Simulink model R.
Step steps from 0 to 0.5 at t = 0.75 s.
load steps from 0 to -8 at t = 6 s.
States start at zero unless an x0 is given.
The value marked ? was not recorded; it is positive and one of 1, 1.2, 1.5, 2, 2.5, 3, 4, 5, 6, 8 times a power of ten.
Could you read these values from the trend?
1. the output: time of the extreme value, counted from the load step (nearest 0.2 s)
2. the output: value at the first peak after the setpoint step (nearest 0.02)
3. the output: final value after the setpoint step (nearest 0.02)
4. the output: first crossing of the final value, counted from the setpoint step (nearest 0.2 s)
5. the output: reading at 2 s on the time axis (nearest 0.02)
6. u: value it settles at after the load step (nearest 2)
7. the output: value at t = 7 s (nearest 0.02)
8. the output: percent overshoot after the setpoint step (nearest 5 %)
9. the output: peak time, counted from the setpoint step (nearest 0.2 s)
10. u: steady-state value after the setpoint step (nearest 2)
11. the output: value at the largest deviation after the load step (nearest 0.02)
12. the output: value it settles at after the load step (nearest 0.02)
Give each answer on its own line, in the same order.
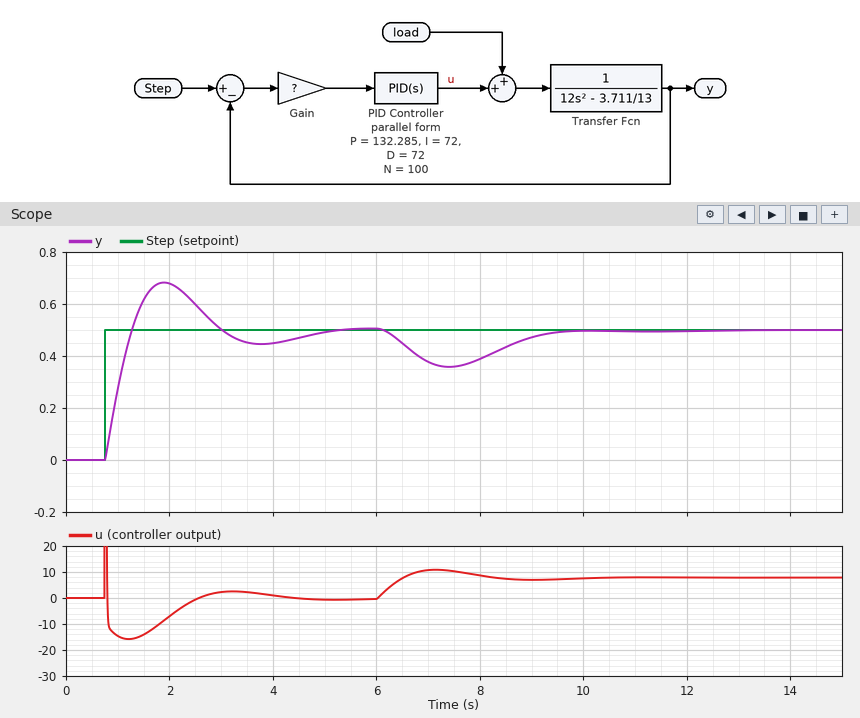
1.4 s
0.68
0.50
0.6 s
0.68
8
0.38
35 %
1.2 s
0
0.36
0.50
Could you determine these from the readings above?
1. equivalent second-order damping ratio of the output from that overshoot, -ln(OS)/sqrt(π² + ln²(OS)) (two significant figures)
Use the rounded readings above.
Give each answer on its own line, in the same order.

0.32
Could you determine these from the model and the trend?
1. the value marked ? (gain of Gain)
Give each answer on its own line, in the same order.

0.4
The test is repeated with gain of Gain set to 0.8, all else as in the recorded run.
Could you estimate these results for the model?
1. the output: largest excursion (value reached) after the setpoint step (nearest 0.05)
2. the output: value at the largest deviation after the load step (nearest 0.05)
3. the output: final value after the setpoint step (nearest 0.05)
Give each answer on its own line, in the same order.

0.60
0.45
0.50
